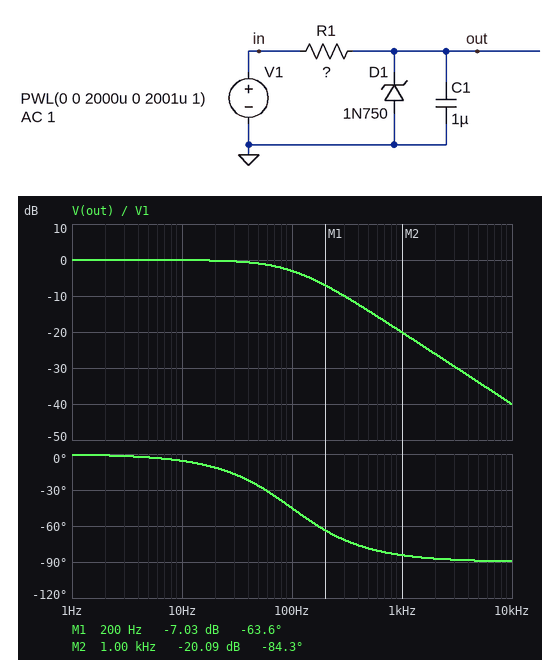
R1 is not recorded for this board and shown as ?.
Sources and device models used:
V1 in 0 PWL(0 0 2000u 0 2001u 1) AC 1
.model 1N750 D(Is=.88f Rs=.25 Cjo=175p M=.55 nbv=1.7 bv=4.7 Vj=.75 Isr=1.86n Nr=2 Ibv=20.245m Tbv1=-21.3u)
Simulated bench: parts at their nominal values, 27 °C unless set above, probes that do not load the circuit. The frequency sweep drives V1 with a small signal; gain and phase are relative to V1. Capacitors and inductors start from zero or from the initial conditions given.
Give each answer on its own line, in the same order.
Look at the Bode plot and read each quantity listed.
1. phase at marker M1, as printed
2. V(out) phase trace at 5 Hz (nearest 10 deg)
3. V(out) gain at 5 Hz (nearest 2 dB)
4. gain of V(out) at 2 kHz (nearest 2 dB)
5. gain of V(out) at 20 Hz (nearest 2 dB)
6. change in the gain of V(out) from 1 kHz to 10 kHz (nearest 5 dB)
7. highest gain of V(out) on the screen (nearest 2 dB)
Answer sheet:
-63.6 deg
0 deg
0 dB
-26 dB
0 dB
-20 dB
0 dB
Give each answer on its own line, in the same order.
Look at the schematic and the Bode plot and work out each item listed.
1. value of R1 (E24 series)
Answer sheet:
1.6 kΩ
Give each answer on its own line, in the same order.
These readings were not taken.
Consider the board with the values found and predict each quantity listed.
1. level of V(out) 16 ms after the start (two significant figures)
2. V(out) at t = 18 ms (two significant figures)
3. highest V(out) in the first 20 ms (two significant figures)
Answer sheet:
1.0 V
1.0 V
1.0 V
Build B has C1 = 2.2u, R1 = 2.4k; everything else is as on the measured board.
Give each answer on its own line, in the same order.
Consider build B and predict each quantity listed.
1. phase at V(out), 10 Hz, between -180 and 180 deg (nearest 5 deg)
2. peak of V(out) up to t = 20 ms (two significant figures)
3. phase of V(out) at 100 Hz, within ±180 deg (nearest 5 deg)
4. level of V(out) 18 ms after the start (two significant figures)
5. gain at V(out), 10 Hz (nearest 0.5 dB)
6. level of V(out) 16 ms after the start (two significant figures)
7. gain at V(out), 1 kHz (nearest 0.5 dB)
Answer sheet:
-20 deg
970 mV
-75 deg
950 mV
-0.5 dB
930 mV
-30.5 dB
